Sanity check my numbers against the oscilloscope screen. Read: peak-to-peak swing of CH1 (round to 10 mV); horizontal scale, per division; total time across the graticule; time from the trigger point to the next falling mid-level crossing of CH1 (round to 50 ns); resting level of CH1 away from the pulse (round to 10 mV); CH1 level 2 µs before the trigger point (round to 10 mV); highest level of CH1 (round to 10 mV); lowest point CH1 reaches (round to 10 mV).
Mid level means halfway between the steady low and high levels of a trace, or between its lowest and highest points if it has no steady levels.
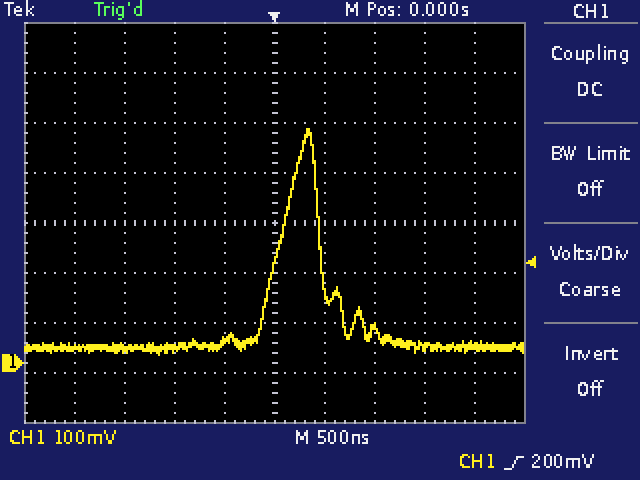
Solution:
450 mV
500 ns
5 µs
450 ns
30 mV
30 mV
470 mV
20 mV
